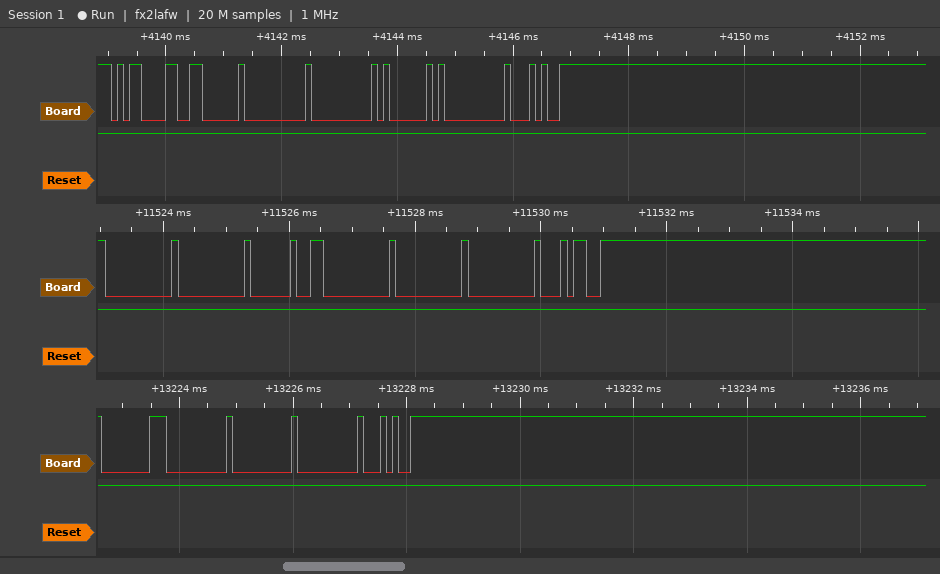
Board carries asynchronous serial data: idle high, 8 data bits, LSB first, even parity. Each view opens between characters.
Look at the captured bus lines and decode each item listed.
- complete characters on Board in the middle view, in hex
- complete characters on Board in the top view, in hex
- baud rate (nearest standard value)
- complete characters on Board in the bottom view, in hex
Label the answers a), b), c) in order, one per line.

a) 00, 00, 20, 00, 00, 00, 34
b) 0D, 06, 00, 00, 81, 00, 94
c) 9600 baud
d) 80, 00, 00, 00, 94
